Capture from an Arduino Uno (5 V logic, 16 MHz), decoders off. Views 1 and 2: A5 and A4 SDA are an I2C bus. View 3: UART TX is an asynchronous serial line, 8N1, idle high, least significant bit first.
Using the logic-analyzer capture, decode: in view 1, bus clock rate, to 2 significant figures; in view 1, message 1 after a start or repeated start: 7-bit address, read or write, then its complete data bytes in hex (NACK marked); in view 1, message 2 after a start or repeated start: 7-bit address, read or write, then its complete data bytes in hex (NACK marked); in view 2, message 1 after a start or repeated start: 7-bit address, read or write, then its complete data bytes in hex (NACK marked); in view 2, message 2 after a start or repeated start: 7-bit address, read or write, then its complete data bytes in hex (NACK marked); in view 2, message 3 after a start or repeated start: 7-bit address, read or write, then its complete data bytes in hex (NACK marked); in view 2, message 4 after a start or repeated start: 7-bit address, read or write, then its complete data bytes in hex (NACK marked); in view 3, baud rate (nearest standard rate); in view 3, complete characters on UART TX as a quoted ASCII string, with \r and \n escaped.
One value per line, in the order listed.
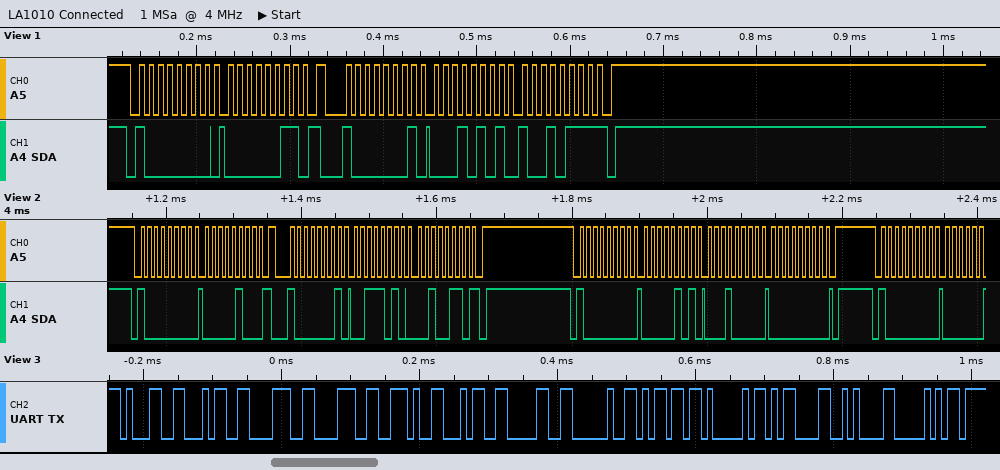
100 kHz
0x40 write: 03
0x40 read: 15 97 NACK
0x40 write: 04
0x40 read: 3A 26 NACK
0x40 write: 05 10 00
0x40 write
115200 baud
"1488.40 mA\r\nP"
